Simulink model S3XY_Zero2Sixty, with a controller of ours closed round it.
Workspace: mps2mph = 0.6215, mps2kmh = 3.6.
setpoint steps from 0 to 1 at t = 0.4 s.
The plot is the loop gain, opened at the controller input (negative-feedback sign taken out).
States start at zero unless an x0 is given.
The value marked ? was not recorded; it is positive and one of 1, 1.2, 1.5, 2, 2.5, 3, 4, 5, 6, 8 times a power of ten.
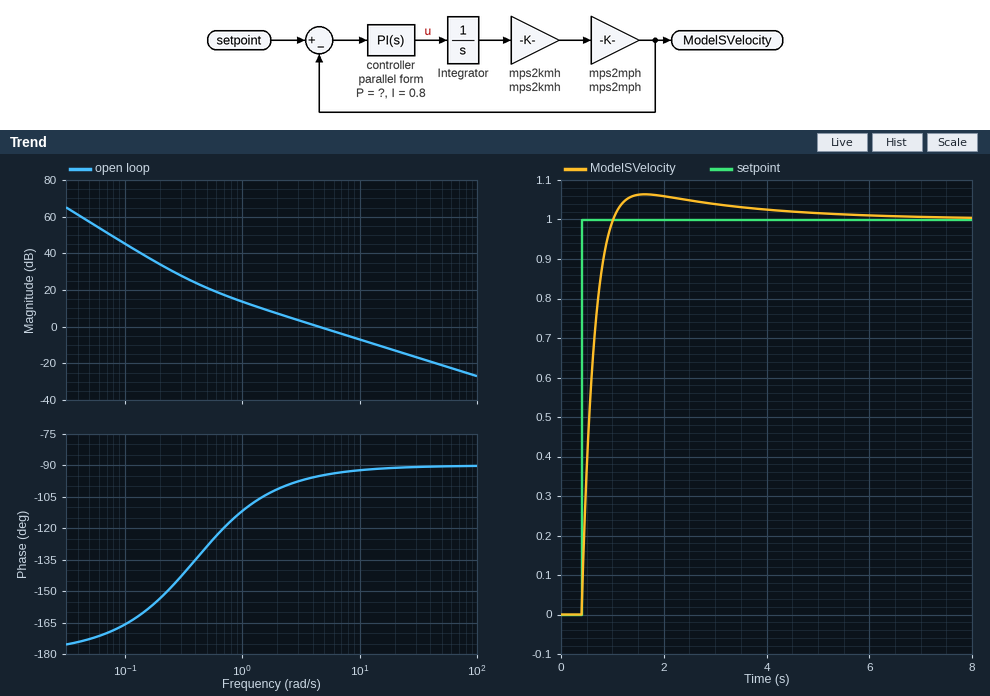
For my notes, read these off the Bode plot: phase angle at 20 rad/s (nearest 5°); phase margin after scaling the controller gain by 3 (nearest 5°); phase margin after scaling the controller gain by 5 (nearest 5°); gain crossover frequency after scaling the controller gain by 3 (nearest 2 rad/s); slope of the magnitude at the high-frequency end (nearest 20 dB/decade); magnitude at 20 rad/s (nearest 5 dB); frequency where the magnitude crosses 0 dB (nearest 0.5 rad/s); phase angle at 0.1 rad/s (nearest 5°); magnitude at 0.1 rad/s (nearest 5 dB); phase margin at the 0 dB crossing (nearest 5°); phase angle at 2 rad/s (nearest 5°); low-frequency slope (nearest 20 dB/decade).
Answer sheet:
-90°
90°
90°
14 rad/s
-20 dB/decade
-15 dB
4.5 rad/s
-165°
45 dB
85°
-100°
-40 dB/decade
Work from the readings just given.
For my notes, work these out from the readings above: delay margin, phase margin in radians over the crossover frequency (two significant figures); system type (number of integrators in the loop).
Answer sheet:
0.33 s
2
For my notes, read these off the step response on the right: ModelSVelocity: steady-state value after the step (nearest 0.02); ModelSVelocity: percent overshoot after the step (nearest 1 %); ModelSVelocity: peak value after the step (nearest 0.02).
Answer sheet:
1.00
6 %
1.06
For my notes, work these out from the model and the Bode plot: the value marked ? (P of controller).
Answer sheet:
2
